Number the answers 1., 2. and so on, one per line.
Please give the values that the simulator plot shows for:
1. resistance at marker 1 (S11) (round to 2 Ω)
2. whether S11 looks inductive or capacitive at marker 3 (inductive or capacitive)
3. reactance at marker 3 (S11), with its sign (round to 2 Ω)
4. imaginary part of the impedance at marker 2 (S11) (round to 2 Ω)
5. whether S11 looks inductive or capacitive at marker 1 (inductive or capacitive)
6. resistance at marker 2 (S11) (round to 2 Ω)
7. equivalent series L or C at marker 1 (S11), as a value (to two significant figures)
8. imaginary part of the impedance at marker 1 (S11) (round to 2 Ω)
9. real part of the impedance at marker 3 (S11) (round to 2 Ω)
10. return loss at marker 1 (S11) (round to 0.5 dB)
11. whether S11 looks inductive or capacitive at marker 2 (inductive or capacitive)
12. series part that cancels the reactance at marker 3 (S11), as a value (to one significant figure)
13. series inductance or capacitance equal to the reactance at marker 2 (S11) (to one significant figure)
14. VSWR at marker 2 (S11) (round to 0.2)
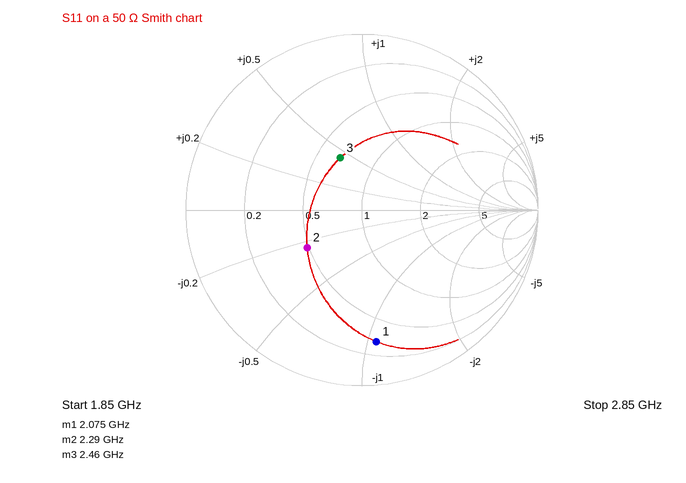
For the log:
1. 16 Ω
2. inductive
3. +22 Ω
4. -12 Ω
5. capacitive
6. 24 Ω
7. 1.4 pF
8. -54 Ω
9. 34 Ω
10. 2.5 dB
11. capacitive
12. 3 pF
13. 6 pF
14. 2.2
